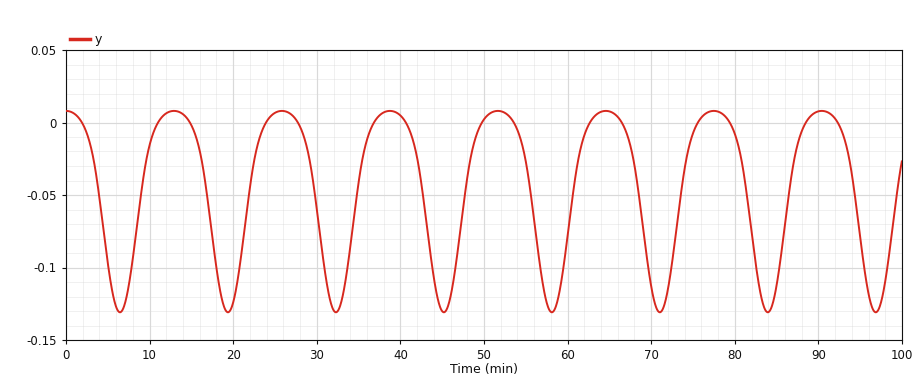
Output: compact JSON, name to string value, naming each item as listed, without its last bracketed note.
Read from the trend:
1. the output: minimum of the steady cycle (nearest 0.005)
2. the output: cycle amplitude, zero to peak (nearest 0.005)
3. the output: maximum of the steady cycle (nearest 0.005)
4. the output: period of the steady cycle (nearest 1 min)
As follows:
{"the output: minimum of the steady cycle": "-0.130", "the output: cycle amplitude, zero to peak": "0.070", "the output: maximum of the steady cycle": "0.010", "the output: period of the steady cycle": "13 min"}
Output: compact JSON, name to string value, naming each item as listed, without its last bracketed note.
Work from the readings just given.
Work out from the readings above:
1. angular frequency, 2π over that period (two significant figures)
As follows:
{"angular frequency, 2π over that period": "0.48 rad/min"}
